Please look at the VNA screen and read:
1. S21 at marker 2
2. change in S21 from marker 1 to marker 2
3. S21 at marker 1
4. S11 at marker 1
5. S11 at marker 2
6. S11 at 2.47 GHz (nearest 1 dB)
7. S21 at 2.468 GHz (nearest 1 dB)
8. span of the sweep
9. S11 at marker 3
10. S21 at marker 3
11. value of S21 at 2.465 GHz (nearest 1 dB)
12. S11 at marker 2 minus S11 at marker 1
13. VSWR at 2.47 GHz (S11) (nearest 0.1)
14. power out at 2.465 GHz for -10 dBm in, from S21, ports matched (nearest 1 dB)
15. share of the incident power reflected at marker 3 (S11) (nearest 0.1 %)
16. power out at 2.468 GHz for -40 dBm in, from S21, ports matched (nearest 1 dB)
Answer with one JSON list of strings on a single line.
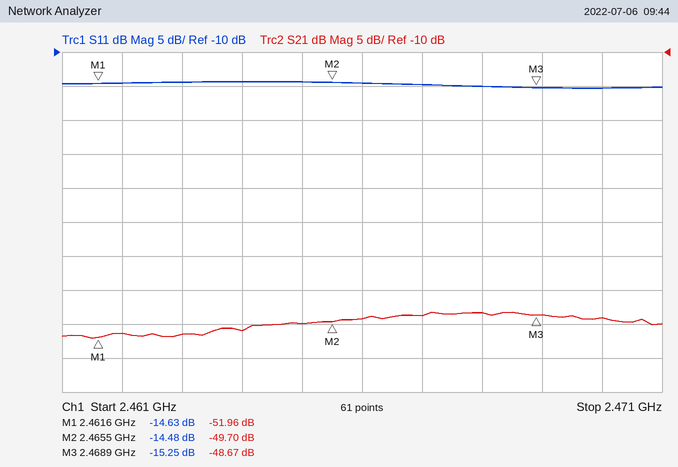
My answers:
["-49.70 dB", "2.26 dB", "-51.96 dB", "-14.63 dB", "-14.48 dB", "-15 dB", "-48 dB", "10 MHz", "-15.25 dB", "-48.67 dB", "-50 dB", "0.15 dB", "1.4", "-60 dBm", "3.0 %", "-88 dBm"]
